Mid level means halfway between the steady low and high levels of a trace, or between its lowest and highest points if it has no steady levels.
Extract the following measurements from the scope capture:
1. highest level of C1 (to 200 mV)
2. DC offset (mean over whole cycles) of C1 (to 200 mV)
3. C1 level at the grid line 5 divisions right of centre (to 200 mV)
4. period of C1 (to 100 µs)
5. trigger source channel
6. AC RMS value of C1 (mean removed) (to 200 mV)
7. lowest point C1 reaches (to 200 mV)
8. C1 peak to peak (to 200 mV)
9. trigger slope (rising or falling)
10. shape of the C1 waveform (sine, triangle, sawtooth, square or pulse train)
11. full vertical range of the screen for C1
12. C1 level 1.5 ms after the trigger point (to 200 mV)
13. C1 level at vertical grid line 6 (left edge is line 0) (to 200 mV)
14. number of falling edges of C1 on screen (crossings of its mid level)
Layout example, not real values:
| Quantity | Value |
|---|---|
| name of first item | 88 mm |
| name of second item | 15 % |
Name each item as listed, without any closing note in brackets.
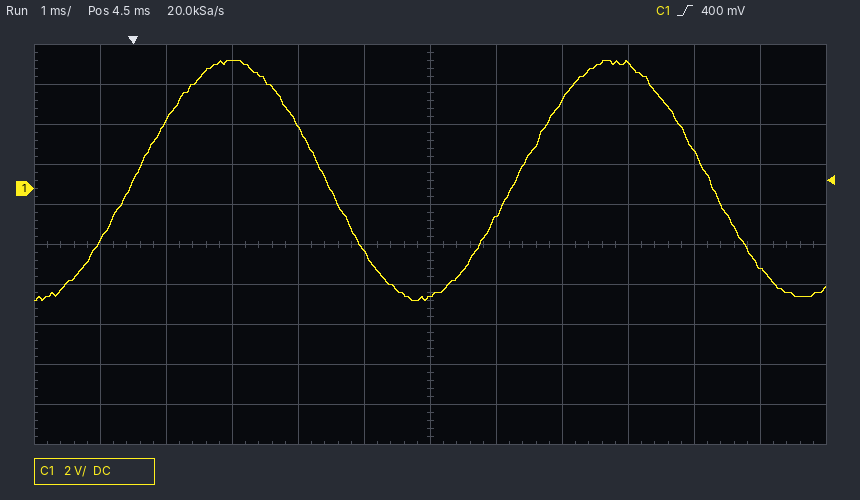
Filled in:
| Quantity | Value |
|---|---|
| highest level of C1 | 6.4 V |
| DC offset (mean over whole cycles) of C1 | 400 mV |
| C1 level at the grid line 5 divisions right of centre | -4.0 V |
| period of C1 | 5.8 ms |
| trigger source channel | C1 |
| AC RMS value of C1 (mean removed) | 4.2 V |
| lowest point C1 reaches | -5.6 V |
| C1 peak to peak | 12.0 V |
| trigger slope | rising |
| shape of the C1 waveform | sine |
| full vertical range of the screen for C1 | 20 V |
| C1 level 1.5 ms after the trigger point | 6.4 V |
| C1 level at vertical grid line 6 (left edge is line 0) | -5.4 V |
| number of falling edges of C1 on screen | 2 |
